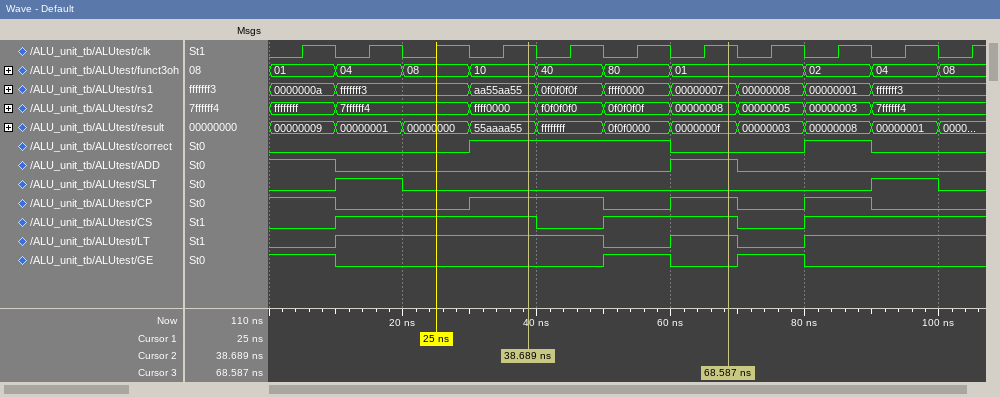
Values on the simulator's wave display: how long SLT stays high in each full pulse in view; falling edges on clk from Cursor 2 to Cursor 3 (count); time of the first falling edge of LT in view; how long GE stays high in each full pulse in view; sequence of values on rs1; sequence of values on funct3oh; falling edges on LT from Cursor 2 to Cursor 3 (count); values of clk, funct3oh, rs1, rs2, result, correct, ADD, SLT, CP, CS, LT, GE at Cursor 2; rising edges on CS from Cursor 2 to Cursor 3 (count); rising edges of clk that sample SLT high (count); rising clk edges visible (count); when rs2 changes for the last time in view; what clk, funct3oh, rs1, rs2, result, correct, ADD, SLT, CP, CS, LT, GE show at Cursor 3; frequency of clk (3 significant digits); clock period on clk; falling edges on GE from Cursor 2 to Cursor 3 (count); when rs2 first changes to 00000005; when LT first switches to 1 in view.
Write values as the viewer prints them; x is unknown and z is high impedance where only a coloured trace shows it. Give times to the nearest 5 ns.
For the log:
10 ns, 10 ns
3
50 ns
10 ns, 10 ns
0000000a, fffffff3, aa55aa55, 0f0f0f0f, ffff0000, 00000007, 00000008, 00000001, fffffff3
01, 04, 08, 10, 40, 80, 01, 02, 04, 08
1
clk=1, funct3oh=10, rs1=aa55aa55, rs2=ffff0000, result=55aaaa55, correct=1, ADD=0, SLT=0, CP=1, CS=1, LT=1, GE=0
1
2
11
90 ns
clk=1, funct3oh=01, rs1=00000007, rs2=00000008, result=0000000f, correct=0, ADD=1, SLT=0, CP=1, CS=1, LT=1, GE=0
100 MHz
10 ns
1
70 ns
10 ns
